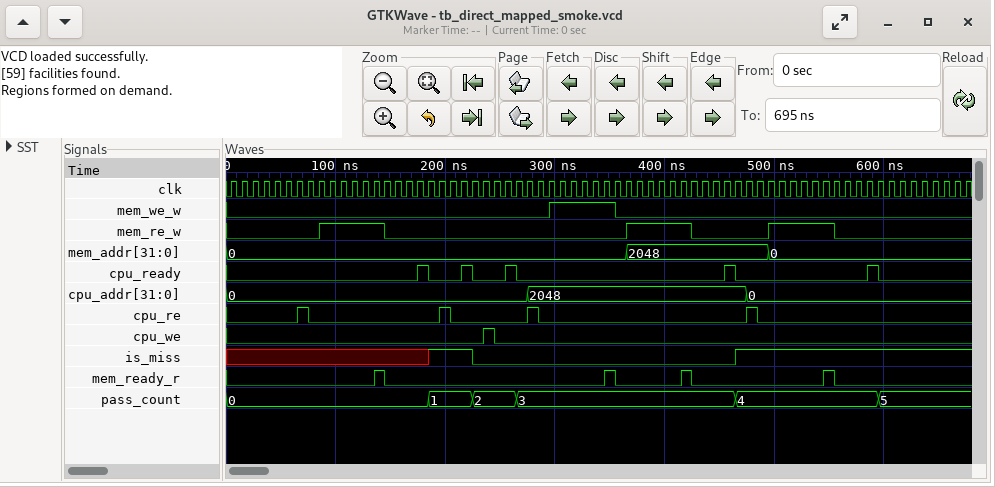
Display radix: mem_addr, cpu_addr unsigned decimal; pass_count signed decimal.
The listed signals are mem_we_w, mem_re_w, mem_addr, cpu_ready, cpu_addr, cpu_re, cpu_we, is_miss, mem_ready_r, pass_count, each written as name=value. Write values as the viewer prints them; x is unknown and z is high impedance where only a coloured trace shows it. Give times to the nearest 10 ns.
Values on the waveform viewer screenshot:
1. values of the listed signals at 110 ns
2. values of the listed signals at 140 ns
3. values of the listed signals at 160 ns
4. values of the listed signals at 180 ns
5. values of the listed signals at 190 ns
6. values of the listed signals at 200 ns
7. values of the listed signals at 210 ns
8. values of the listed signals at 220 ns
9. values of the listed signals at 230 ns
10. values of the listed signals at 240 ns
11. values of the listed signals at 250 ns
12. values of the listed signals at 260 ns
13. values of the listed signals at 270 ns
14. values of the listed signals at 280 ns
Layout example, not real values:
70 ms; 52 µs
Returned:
mem_we_w=0, mem_re_w=1, mem_addr=0, cpu_ready=0, cpu_addr=0, cpu_re=0, cpu_we=0, is_miss=x, mem_ready_r=0, pass_count=0; mem_we_w=0, mem_re_w=1, mem_addr=0, cpu_ready=0, cpu_addr=0, cpu_re=0, cpu_we=0, is_miss=x, mem_ready_r=1, pass_count=0; mem_we_w=0, mem_re_w=0, mem_addr=0, cpu_ready=0, cpu_addr=0, cpu_re=0, cpu_we=0, is_miss=x, mem_ready_r=0, pass_count=0; mem_we_w=0, mem_re_w=0, mem_addr=0, cpu_ready=1, cpu_addr=0, cpu_re=0, cpu_we=0, is_miss=x, mem_ready_r=0, pass_count=0; mem_we_w=0, mem_re_w=0, mem_addr=0, cpu_ready=0, cpu_addr=0, cpu_re=0, cpu_we=0, is_miss=1, mem_ready_r=0, pass_count=1; mem_we_w=0, mem_re_w=0, mem_addr=0, cpu_ready=0, cpu_addr=0, cpu_re=1, cpu_we=0, is_miss=1, mem_ready_r=0, pass_count=1; mem_we_w=0, mem_re_w=0, mem_addr=0, cpu_ready=0, cpu_addr=0, cpu_re=0, cpu_we=0, is_miss=1, mem_ready_r=0, pass_count=1; mem_we_w=0, mem_re_w=0, mem_addr=0, cpu_ready=1, cpu_addr=0, cpu_re=0, cpu_we=0, is_miss=1, mem_ready_r=0, pass_count=1; mem_we_w=0, mem_re_w=0, mem_addr=0, cpu_ready=0, cpu_addr=0, cpu_re=0, cpu_we=0, is_miss=0, mem_ready_r=0, pass_count=2; mem_we_w=0, mem_re_w=0, mem_addr=0, cpu_ready=0, cpu_addr=0, cpu_re=0, cpu_we=1, is_miss=0, mem_ready_r=0, pass_count=2; mem_we_w=0, mem_re_w=0, mem_addr=0, cpu_ready=0, cpu_addr=0, cpu_re=0, cpu_we=0, is_miss=0, mem_ready_r=0, pass_count=2; mem_we_w=0, mem_re_w=0, mem_addr=0, cpu_ready=1, cpu_addr=0, cpu_re=0, cpu_we=0, is_miss=0, mem_ready_r=0, pass_count=2; mem_we_w=0, mem_re_w=0, mem_addr=0, cpu_ready=0, cpu_addr=0, cpu_re=0, cpu_we=0, is_miss=0, mem_ready_r=0, pass_count=3; mem_we_w=0, mem_re_w=0, mem_addr=0, cpu_ready=0, cpu_addr=2048, cpu_re=1, cpu_we=0, is_miss=0, mem_ready_r=0, pass_count=3
